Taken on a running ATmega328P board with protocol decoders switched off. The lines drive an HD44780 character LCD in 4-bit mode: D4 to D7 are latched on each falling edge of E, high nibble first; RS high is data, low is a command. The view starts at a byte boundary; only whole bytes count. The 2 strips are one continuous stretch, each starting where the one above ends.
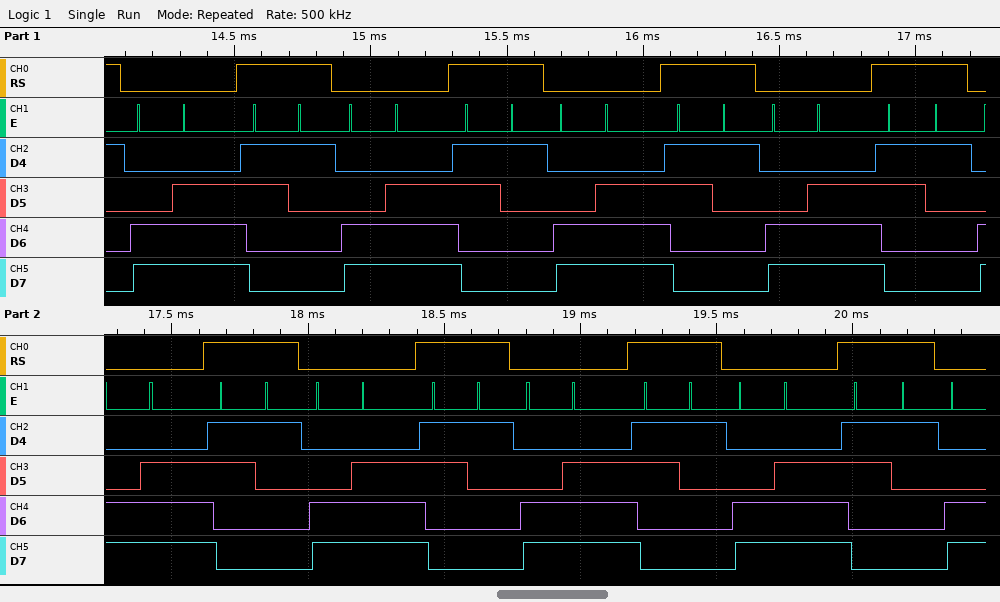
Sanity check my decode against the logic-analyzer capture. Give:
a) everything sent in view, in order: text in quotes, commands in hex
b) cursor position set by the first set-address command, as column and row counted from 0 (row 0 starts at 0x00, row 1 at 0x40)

0xCE "1" 0xCE "1" 0xCE "1" 0xCE "1" 0xCE "1" 0xCE "1" 0xCE "1" 0xCE "1"
column 14, row 1
